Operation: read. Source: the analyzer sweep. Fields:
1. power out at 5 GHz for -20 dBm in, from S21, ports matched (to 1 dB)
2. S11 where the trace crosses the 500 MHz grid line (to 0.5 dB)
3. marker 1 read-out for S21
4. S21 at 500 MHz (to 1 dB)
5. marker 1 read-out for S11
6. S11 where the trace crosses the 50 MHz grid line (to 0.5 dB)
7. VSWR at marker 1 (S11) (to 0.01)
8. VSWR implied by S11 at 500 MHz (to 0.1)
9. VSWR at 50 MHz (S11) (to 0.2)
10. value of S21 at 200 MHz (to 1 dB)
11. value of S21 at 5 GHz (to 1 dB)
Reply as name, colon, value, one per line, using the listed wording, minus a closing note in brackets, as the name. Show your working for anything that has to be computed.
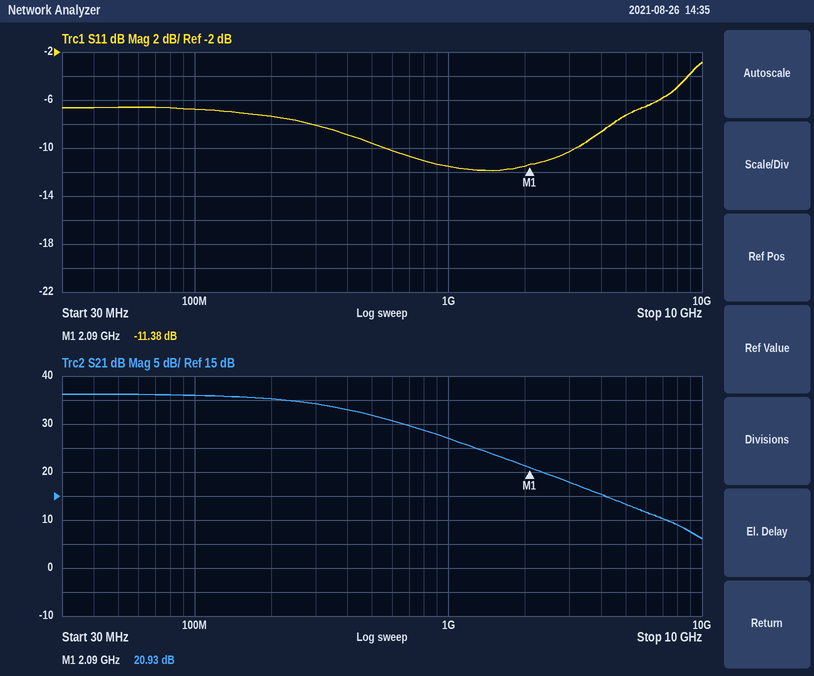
power out at 5 GHz for -20 dBm in, from S21, ports matched: -20 dBm + (13 dB) = -7 dBm
S11 where the trace crosses the 500 MHz grid line: -9.5 dB
marker 1 read-out for S21: 20.93 dB
S21 at 500 MHz: 32 dB
marker 1 read-out for S11: -11.38 dB
S11 where the trace crosses the 50 MHz grid line: -6.5 dB
VSWR at marker 1 (S11): (1 + 0.2698)/(1 − 0.2698) ≈ 1.74
VSWR implied by S11 at 500 MHz: |Γ| = 10^(-9.5/20) = 0.3350; VSWR = (1 + 0.3350)/(1 − 0.3350) ≈ 2.0
VSWR at 50 MHz (S11): |Γ| = 10^(-6.5/20) = 0.4732; VSWR = (1 + 0.4732)/(1 − 0.4732) ≈ 2.8
value of S21 at 200 MHz: 35 dB
value of S21 at 5 GHz: 13 dB
